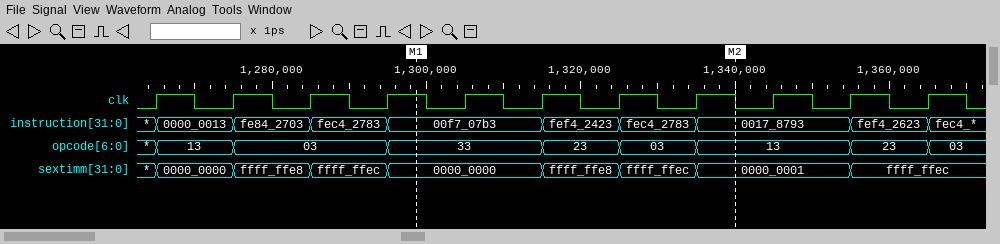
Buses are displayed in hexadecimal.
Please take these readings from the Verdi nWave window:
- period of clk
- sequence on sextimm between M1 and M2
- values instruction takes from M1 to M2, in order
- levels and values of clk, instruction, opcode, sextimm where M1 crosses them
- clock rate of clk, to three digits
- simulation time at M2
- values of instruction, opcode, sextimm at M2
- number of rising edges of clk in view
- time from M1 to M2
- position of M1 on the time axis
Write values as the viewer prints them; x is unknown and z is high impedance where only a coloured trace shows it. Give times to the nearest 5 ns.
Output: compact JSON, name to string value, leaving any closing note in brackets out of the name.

{"period of clk": "10 ns", "sequence on sextimm between M1 and M2": "0000_0000, ffff_ffe8, ffff_ffec, 0000_0001", "values instruction takes from M1 to M2, in order": "00f7_07b3, fef4_2423, fec4_2783, 0017_8793", "levels and values of clk, instruction, opcode, sextimm where M1 crosses them": "clk=1, instruction=00f7_07b3, opcode=33, sextimm=0000_0000", "clock rate of clk, to three digits": "100 MHz", "simulation time at M2": "1340 ns", "values of instruction, opcode, sextimm at M2": "instruction=0017_8793, opcode=13, sextimm=0000_0001", "number of rising edges of clk in view": "11", "time from M1 to M2": "40 ns", "position of M1 on the time axis": "1300 ns"}
